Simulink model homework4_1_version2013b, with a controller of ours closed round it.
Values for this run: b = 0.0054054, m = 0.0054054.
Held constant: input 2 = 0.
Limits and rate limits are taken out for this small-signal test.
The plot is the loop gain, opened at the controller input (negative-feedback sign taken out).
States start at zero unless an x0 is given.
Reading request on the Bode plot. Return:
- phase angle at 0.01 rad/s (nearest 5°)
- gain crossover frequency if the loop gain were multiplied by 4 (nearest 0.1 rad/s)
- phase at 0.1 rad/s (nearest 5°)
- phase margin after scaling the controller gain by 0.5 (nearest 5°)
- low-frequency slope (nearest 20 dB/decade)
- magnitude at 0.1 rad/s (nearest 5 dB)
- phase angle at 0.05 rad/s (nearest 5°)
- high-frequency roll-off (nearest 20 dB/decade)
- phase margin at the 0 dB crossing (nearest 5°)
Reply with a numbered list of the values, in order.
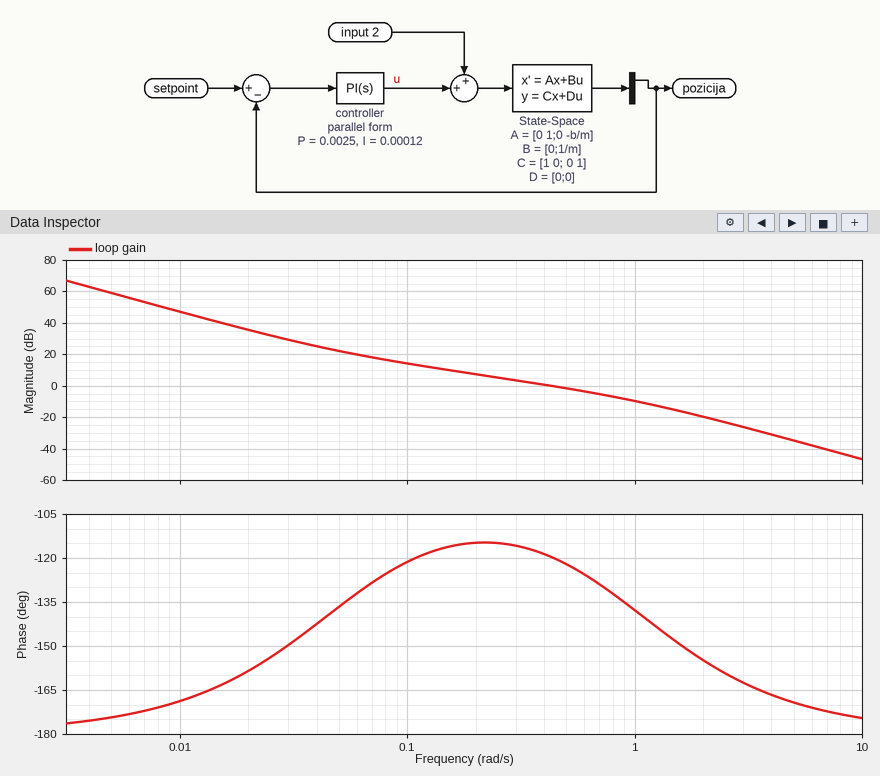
1. -170°
2. 1.2 rad/s
3. -120°
4. 65°
5. -40 dB/decade
6. 15 dB
7. -135°
8. -40 dB/decade
9. 60°
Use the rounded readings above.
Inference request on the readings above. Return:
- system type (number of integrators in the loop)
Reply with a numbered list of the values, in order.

1. 2
